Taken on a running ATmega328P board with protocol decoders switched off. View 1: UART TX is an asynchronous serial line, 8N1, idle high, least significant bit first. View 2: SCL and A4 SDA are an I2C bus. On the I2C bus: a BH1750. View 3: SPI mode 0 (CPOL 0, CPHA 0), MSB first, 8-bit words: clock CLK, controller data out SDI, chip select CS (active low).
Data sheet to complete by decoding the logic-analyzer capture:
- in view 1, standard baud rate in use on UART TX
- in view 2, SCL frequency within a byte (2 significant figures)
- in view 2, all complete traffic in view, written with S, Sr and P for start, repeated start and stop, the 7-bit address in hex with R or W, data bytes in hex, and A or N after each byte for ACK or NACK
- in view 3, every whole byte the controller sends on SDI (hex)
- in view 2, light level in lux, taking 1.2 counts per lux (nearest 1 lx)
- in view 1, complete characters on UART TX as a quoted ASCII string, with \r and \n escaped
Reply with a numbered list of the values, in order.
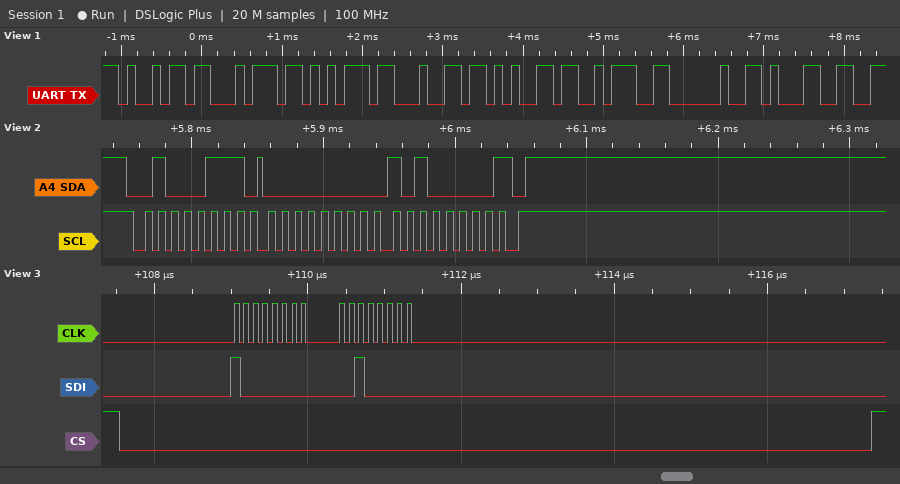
1. 9600 baud
2. 100 kHz
3. S 23R A 00 A A0 N P
4. 80 20
5. 133 lx
6. "itude: 1"
